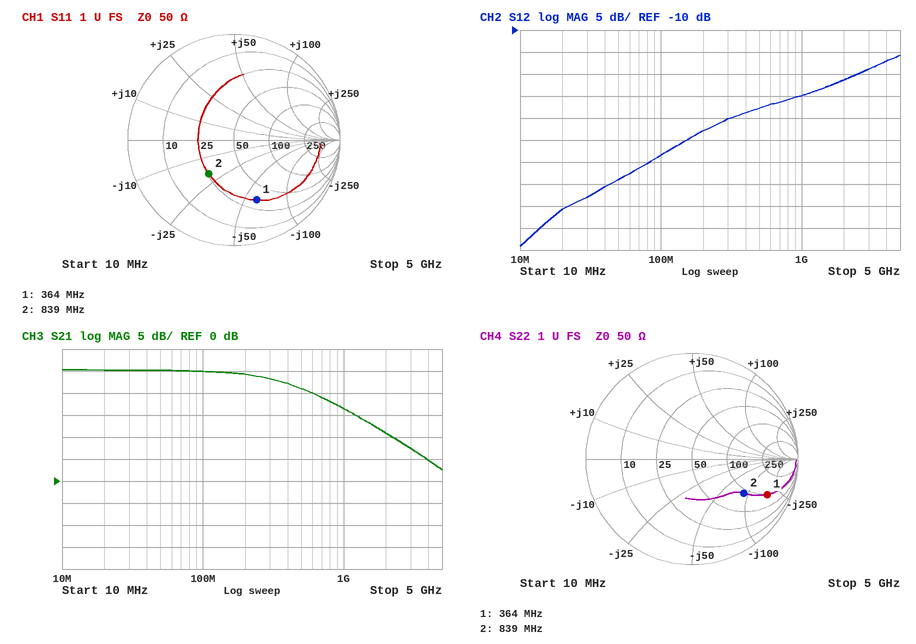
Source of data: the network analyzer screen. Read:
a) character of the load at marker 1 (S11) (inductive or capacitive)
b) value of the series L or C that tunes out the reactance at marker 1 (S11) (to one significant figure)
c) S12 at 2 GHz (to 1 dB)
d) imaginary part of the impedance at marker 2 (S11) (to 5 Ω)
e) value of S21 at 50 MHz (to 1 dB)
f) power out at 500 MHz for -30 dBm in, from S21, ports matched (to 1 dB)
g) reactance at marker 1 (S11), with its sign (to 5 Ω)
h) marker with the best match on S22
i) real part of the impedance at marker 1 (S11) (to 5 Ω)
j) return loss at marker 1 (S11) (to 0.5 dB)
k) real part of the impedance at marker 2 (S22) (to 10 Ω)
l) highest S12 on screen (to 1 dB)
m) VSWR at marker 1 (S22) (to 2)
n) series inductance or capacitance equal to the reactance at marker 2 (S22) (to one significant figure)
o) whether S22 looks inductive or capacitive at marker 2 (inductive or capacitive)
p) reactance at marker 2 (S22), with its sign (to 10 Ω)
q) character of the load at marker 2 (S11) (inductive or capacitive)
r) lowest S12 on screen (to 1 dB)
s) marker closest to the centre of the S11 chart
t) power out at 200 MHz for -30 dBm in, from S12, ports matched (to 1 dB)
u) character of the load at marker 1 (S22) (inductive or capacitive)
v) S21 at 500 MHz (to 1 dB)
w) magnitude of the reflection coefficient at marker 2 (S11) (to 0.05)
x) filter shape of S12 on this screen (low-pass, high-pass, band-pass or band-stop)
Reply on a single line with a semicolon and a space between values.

capacitive; 30 nH; -21 dB; -20 Ω; 25 dB; -9 dBm; -60 Ω; marker 2; 35 Ω; 4.5 dB; 90 Ω; -16 dB; 8; 2 pF; capacitive; -90 Ω; capacitive; -59 dB; marker 2; -63 dBm; capacitive; 21 dB; 0.40; high-pass
